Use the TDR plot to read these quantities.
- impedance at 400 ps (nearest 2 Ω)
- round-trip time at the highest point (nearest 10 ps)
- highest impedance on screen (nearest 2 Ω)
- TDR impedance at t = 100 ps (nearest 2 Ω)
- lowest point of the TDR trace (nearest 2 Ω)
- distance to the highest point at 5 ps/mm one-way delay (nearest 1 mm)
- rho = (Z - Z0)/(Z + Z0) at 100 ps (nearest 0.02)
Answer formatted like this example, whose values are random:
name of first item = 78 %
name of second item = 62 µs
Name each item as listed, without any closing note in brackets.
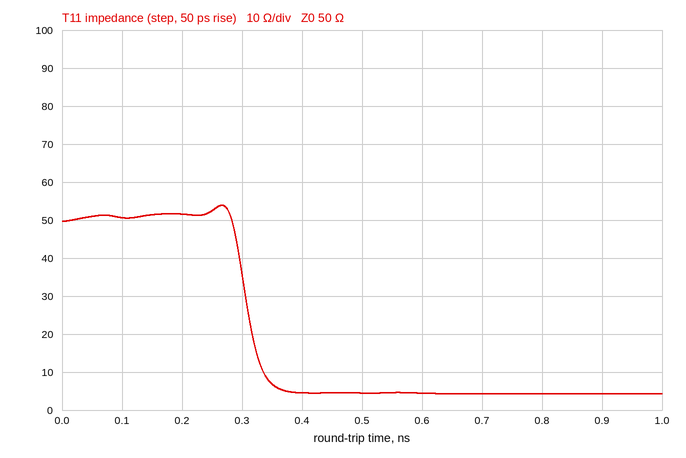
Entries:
impedance at 400 ps = 4 Ω
round-trip time at the highest point = 270 ps
highest impedance on screen = 54 Ω
TDR impedance at t = 100 ps = 50 Ω
lowest point of the TDR trace = 4 Ω
distance to the highest point at 5 ps/mm one-way delay = 27 mm
rho = (Z - Z0)/(Z + Z0) at 100 ps = 0.00
